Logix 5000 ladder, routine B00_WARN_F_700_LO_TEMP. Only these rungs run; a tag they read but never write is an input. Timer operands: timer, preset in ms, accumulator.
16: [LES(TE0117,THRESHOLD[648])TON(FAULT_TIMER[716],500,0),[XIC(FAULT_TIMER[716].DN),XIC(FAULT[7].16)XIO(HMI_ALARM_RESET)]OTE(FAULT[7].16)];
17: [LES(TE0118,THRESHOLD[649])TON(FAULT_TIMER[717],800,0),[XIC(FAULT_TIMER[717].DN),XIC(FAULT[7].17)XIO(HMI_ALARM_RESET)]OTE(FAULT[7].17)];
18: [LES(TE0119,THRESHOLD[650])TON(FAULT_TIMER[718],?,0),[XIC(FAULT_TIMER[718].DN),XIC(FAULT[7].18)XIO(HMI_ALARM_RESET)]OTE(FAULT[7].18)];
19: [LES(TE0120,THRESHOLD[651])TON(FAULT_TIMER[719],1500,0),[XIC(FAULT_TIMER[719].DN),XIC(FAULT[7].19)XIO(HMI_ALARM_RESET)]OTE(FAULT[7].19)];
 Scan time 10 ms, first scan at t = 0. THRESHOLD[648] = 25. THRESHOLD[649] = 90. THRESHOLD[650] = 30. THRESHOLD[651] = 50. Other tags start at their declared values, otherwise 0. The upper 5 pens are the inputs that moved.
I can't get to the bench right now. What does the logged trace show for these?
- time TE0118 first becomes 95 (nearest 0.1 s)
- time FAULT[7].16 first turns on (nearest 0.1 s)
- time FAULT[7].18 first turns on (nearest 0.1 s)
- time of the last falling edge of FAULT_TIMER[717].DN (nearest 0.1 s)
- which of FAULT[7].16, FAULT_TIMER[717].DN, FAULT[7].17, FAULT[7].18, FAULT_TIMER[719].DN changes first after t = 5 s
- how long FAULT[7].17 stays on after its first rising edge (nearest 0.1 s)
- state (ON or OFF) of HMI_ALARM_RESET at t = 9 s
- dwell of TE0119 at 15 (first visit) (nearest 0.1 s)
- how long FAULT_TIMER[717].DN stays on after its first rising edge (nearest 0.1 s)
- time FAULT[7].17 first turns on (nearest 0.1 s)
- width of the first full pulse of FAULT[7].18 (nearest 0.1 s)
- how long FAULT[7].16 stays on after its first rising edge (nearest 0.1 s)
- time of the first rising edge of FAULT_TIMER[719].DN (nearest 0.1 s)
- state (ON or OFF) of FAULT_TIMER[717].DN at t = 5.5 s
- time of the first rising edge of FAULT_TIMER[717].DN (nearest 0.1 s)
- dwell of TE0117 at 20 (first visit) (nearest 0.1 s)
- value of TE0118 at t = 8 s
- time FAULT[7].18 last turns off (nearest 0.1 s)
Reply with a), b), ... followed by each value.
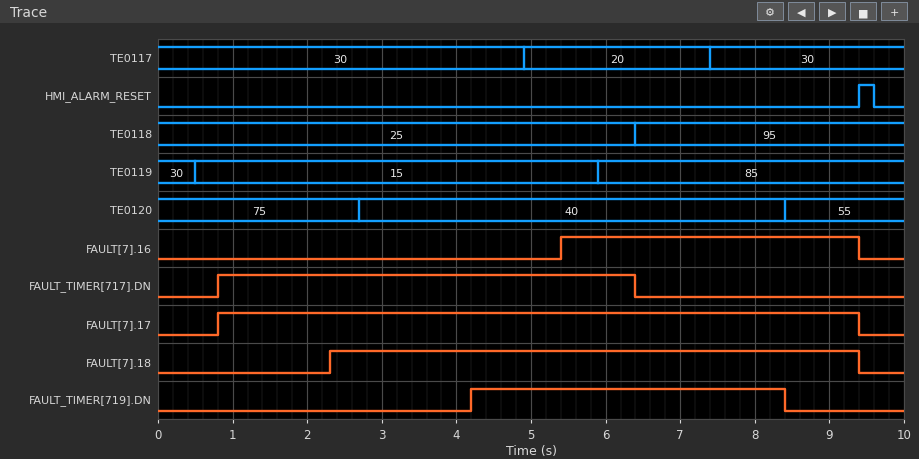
a) 6.4 s
b) 5.4 s
c) 2.3 s
d) 6.4 s
e) FAULT[7].16
f) 8.6 s
g) OFF
h) 5.4 s
i) 5.6 s
j) 0.8 s
k) 7.1 s
l) 4.0 s
m) 4.2 s
n) ON
o) 0.8 s
p) 2.5 s
q) 95
r) 9.4 s
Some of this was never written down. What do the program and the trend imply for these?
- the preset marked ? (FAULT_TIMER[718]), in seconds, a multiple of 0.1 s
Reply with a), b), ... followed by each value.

a) 1.8 s
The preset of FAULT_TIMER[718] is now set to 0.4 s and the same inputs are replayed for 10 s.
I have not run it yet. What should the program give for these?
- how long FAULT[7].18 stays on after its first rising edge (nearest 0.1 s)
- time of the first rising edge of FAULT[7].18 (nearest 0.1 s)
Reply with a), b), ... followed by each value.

a) 8.5 s
b) 0.9 s
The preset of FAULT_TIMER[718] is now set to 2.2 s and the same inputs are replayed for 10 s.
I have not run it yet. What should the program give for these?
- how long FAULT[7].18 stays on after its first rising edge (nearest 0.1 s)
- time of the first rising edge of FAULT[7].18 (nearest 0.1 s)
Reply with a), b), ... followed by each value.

a) 6.7 s
b) 2.7 s
